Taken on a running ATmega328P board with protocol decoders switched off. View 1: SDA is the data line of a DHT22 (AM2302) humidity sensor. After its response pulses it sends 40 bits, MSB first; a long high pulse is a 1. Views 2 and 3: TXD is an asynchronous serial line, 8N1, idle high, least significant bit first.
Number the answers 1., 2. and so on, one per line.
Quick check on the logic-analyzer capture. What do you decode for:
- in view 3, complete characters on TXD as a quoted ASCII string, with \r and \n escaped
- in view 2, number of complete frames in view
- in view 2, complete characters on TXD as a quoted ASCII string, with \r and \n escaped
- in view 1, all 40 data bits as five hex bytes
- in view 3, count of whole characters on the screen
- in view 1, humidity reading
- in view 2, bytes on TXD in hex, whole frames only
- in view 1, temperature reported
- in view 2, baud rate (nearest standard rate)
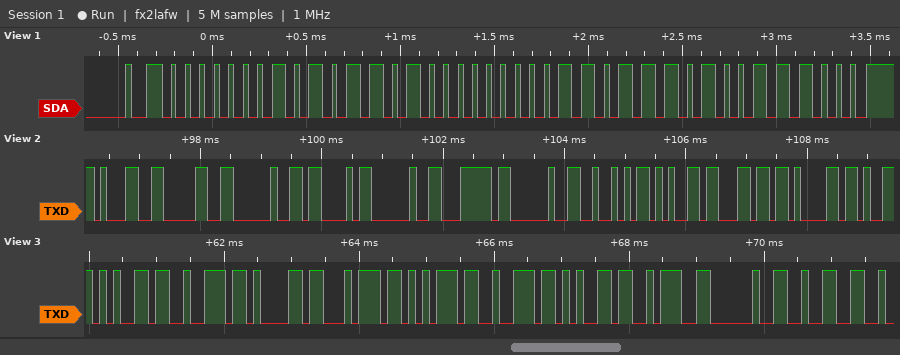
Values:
1. "erature: 2"
2. 11
3. "10 C | Rela"
4. 01 5A 00 DD 38
5. 10
6. 34.6 %
7. 0x31 0x30 0x20 0x43 0x20 0x7C 0x20 0x52 0x65 0x6C 0x61
8. 22.1 °C
9. 9600 baud
